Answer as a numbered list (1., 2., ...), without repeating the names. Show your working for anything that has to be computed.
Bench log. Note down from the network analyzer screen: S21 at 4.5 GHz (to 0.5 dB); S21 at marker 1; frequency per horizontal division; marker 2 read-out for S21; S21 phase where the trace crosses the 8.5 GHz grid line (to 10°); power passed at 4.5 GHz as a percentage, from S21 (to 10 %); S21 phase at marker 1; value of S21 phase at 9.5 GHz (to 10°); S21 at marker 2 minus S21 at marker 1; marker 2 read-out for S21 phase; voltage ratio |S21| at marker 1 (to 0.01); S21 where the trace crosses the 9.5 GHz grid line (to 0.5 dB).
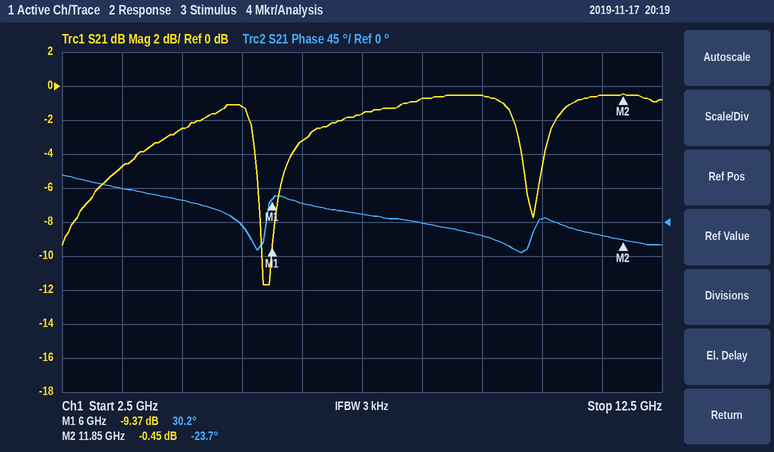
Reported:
1. -2.5 dB
2. -9.37 dB
3. 1 GHz
4. -0.45 dB
5. 0°
6. 10^(-2.5/10) ≈ 56.2 %, so 60 % to the nearest 10 %
7. 30.2°
8. -20°
9. -0.45 − (-9.37) = 8.92 dB
10. -23.7°
11. 10^(-9.37/20) ≈ 0.34
12. -0.5 dB
